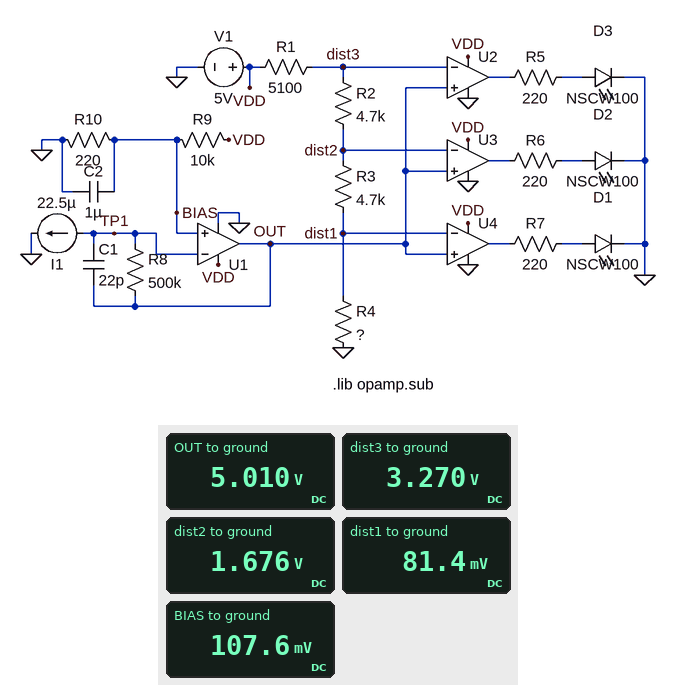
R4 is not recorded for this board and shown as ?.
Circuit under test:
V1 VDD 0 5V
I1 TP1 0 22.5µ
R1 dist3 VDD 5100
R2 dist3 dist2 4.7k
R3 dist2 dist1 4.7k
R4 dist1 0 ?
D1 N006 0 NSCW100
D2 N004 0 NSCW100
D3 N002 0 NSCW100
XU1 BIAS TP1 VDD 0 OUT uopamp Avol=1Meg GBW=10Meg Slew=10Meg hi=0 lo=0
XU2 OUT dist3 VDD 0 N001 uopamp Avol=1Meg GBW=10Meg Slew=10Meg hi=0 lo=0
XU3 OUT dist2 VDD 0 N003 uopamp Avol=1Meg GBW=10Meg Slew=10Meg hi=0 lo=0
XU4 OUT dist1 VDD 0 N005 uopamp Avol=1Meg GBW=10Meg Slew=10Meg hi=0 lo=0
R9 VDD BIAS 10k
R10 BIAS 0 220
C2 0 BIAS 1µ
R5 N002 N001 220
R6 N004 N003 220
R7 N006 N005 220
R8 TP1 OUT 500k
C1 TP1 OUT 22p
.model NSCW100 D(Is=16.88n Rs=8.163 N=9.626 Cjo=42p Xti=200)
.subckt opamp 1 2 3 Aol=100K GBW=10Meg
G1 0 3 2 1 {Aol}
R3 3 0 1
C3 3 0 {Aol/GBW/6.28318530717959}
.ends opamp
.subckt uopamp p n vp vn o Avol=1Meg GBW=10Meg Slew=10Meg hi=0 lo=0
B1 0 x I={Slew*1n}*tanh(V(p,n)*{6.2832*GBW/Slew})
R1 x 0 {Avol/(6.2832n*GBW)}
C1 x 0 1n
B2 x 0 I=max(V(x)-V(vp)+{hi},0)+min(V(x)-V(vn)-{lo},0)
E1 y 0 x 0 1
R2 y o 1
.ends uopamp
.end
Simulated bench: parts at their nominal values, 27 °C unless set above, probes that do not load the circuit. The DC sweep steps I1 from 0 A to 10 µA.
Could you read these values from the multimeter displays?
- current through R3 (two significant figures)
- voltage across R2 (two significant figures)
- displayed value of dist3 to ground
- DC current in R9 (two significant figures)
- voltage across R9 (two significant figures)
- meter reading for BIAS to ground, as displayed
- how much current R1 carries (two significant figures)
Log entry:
340 µA
1.6 V
3.270 V
490 µA
4.9 V
107.6 mV
340 µA
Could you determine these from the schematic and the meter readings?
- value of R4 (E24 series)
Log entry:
240 Ω
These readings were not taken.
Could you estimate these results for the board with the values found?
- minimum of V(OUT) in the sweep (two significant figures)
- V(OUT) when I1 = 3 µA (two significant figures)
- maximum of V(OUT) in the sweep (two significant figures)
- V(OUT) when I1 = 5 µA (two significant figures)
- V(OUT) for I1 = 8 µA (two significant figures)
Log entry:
110 mV
1.6 V
5.0 V
2.6 V
4.1 V
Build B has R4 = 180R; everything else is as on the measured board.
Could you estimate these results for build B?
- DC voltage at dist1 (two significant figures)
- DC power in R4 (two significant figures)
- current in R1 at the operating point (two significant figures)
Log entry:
61 mV
21 µW
340 µA
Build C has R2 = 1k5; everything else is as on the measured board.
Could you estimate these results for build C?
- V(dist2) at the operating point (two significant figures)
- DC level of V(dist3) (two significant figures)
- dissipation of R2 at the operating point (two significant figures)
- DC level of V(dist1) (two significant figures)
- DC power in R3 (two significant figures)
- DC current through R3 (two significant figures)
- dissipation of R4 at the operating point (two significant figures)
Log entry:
2.1 V
2.8 V
280 µW
100 mV
880 µW
430 µA
45 µW
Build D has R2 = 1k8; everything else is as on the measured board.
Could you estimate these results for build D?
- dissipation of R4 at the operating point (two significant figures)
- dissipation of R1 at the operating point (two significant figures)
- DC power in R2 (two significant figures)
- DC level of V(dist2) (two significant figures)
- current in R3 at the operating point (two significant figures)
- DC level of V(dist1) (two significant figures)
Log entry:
43 µW
910 µW
320 µW
2.1 V
420 µA
100 mV
